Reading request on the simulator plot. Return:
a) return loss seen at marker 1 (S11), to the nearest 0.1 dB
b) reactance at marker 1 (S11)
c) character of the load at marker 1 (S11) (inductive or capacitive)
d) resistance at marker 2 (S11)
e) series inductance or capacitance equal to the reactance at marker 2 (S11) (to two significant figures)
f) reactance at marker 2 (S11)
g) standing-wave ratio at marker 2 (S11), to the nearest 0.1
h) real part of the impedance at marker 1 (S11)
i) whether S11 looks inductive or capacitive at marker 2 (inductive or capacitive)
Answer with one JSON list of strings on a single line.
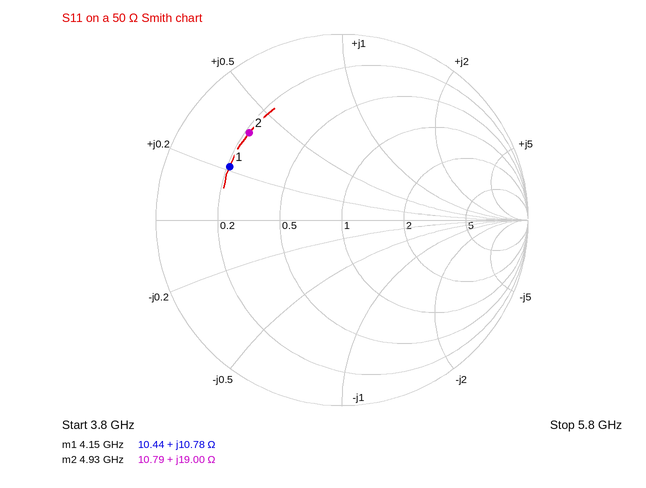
["3.5 dB", "+10.78 Ω", "inductive", "10.79 Ω", "610 pH", "+19.00 Ω", "5.3", "10.44 Ω", "inductive"]
